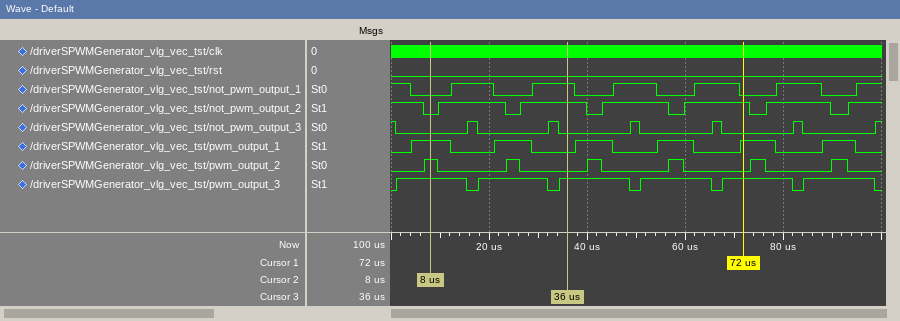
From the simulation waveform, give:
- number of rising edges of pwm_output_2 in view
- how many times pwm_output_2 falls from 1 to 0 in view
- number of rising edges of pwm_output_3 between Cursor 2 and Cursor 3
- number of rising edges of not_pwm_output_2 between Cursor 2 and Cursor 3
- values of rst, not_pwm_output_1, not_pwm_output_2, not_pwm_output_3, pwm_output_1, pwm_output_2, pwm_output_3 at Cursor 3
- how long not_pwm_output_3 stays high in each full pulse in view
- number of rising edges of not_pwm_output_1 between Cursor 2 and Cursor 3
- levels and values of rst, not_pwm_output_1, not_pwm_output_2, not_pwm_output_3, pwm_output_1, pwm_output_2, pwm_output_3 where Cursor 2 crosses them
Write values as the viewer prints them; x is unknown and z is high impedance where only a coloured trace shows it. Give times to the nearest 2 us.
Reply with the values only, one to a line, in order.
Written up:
6
6
2
2
rst=0, not_pwm_output_1=1, not_pwm_output_2=1, not_pwm_output_3=0, pwm_output_1=0, pwm_output_2=0, pwm_output_3=1
2 us, 2 us, 2 us, 2 us, 2 us
2
rst=0, not_pwm_output_1=0, not_pwm_output_2=0, not_pwm_output_3=0, pwm_output_1=1, pwm_output_2=1, pwm_output_3=1
